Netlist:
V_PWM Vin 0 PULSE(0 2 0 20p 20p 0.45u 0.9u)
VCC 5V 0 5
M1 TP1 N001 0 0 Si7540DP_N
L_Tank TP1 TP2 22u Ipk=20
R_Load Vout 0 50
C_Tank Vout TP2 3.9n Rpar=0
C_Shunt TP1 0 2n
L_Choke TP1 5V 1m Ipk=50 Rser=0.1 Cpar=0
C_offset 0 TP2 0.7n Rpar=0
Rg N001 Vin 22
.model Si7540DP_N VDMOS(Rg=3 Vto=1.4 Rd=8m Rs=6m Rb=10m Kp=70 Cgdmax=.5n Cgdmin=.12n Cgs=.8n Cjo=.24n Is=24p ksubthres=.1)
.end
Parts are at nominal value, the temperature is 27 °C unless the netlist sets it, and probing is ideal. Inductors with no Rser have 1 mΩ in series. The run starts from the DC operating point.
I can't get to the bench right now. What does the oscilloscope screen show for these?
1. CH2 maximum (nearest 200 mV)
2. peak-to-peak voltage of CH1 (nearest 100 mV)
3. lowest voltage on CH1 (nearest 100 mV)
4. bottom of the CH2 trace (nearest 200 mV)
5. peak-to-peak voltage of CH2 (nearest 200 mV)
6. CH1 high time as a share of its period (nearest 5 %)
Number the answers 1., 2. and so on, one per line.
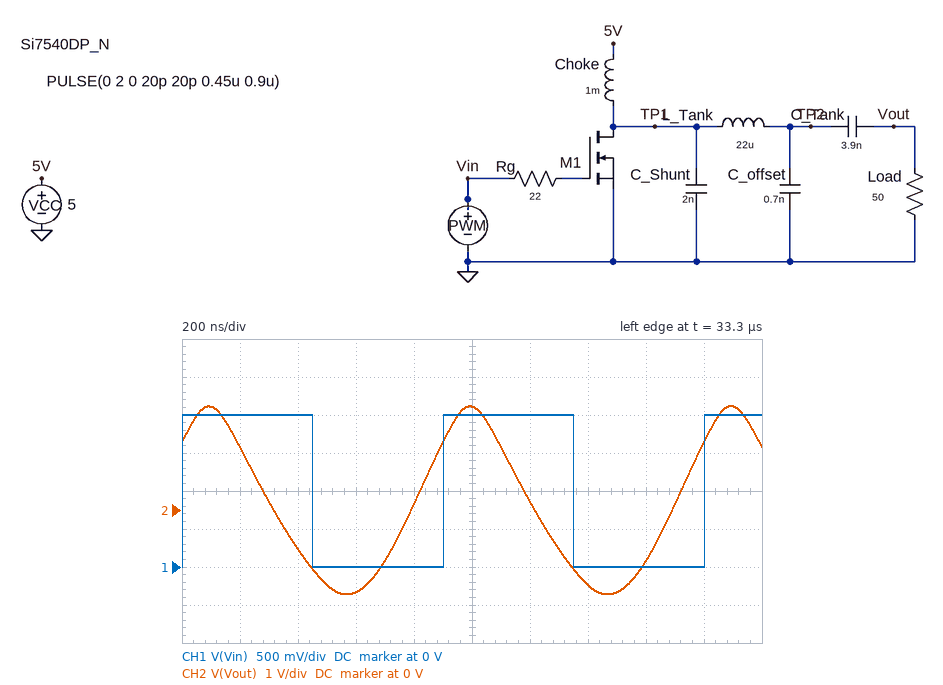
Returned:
1. 2.8 V
2. 2.0 V
3. 0 V
4. -2.2 V
5. 5.0 V
6. 50 %
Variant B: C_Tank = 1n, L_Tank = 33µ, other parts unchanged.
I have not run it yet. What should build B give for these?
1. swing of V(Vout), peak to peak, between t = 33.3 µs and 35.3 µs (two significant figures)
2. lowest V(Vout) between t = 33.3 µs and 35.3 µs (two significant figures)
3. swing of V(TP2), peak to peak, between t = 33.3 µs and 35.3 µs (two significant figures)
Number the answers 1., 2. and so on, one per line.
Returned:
1. 2.9 V
2. -1.3 V
3. 8.2 V
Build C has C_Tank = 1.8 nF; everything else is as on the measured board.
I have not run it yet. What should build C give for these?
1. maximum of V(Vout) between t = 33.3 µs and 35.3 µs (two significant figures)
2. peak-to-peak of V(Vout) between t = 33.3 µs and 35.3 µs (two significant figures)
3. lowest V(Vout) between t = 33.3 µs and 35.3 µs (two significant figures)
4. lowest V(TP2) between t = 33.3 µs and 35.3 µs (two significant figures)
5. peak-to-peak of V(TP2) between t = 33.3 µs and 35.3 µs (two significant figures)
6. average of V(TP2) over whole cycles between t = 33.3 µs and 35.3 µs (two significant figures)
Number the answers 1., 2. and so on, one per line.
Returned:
1. 2.9 V
2. 5.3 V
3. -2.5 V
4. 160 mV
5. 9.4 V
6. 5.0 V
